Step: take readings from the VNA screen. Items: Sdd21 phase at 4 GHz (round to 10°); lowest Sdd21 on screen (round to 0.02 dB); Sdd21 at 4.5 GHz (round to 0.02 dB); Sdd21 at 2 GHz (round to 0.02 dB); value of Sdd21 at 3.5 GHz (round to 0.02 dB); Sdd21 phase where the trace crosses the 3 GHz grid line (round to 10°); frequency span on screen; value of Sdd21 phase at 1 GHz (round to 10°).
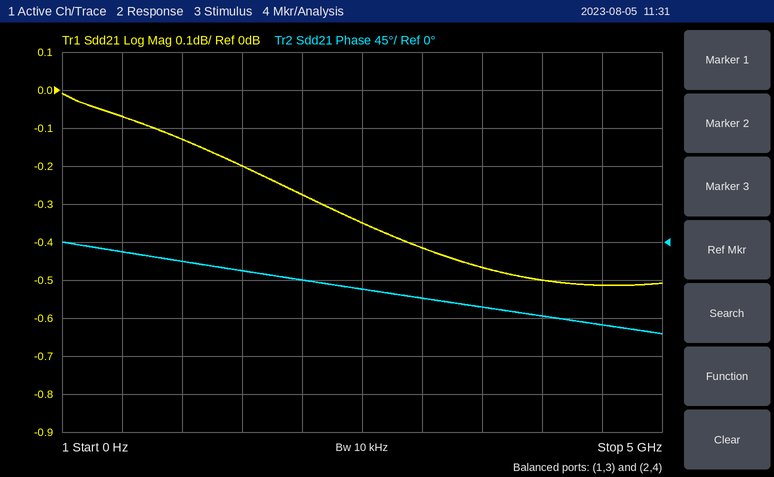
-90°
-0.52 dB
-0.52 dB
-0.28 dB
-0.46 dB
-70°
5 GHz
-20°
